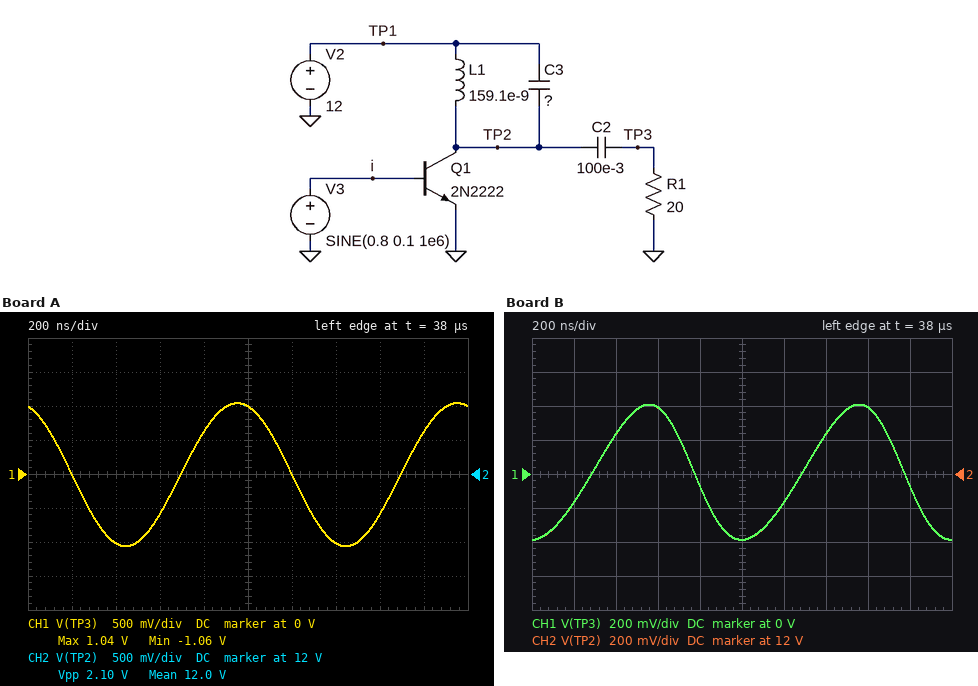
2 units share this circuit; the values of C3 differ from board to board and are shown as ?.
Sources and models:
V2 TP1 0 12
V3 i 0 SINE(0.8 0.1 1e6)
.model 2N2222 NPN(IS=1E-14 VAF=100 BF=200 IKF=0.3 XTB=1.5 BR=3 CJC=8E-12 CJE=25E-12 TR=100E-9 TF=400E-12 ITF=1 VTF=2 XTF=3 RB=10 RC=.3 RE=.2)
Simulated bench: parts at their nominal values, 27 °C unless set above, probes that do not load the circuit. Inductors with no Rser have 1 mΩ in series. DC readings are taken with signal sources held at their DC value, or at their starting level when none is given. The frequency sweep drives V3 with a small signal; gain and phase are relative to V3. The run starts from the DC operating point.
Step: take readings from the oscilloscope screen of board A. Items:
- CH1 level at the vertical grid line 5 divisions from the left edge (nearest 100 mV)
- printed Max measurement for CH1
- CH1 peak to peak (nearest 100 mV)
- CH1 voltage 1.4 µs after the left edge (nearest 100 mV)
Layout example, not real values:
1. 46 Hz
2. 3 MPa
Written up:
1. 1.0 V
2. 1.04 V
3. 2.1 V
4. -1.0 V
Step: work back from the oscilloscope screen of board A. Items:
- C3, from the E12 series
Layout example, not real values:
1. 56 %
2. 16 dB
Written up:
1. 180 nF
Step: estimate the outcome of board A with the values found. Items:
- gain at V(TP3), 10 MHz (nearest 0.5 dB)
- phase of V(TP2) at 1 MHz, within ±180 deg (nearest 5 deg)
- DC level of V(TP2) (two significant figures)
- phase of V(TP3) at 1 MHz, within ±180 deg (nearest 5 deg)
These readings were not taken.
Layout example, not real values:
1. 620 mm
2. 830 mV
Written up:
1. -17.5 dB
2. 110 deg
3. 12 V
4. 110 deg
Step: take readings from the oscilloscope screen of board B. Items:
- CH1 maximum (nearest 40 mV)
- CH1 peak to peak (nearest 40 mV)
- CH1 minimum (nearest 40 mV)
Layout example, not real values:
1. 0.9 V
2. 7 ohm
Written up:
1. 400 mV
2. 800 mV
3. -400 mV
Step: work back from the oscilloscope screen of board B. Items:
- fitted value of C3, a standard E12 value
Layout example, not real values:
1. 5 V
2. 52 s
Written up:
1. 100 nF
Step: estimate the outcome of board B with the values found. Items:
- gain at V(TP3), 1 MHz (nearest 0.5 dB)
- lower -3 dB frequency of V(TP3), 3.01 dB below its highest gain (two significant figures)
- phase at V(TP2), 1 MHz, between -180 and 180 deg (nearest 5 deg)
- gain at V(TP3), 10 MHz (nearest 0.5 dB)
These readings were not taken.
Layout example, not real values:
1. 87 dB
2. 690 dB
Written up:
1. 13.0 dB
2. 1.2 MHz
3. -100 deg
4. -12.5 dB
